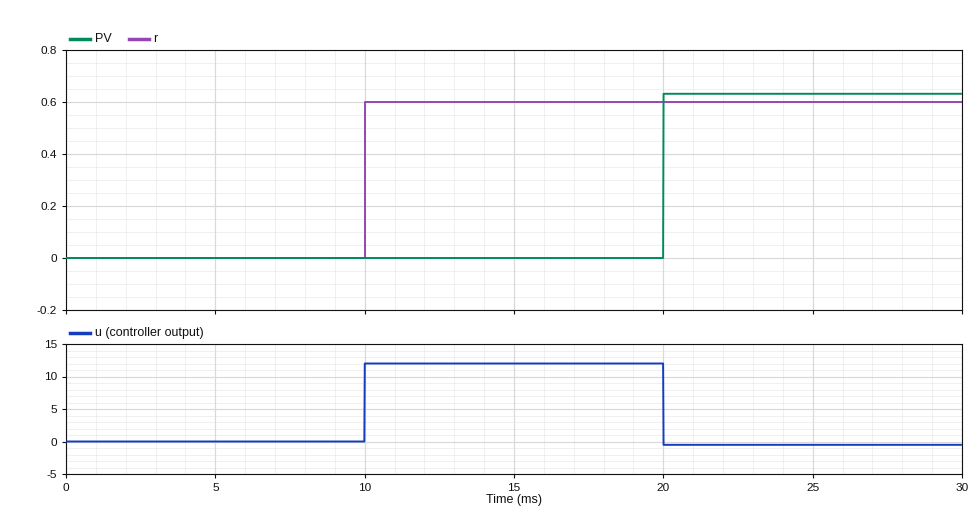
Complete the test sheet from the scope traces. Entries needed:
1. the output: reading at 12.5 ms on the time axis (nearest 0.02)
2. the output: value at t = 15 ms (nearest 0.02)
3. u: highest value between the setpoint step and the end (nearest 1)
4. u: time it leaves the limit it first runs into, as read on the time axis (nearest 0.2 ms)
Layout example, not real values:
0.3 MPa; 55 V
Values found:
0.00; 0.00; 12; 20.0 ms
